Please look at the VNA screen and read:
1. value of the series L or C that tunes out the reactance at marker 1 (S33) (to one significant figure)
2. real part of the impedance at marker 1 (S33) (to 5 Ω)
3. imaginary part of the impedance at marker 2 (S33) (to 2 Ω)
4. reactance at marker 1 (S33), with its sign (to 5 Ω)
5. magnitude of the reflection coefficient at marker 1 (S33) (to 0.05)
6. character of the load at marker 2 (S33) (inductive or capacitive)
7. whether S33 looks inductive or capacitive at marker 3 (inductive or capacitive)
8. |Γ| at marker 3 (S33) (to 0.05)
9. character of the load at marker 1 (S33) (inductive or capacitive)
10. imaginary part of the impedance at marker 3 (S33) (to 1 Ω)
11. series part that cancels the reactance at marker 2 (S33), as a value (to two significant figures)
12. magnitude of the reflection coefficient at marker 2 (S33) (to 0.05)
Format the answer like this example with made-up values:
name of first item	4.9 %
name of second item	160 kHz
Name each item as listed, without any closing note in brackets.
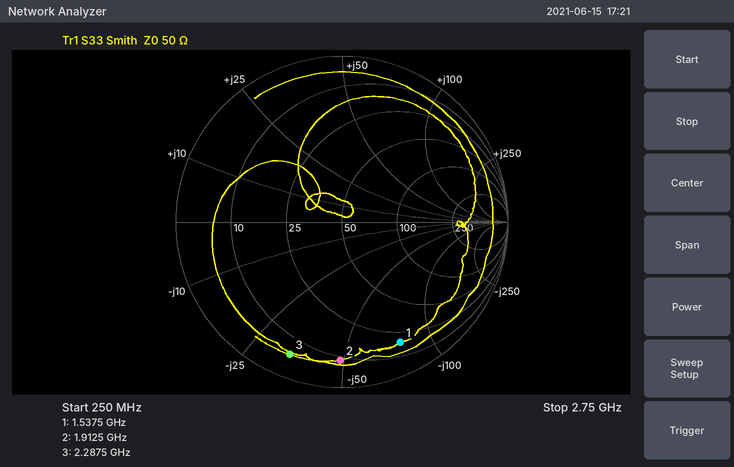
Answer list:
value of the series L or C that tunes out the reactance at marker 1 (S33)	8 nH
real part of the impedance at marker 1 (S33)	20 Ω
imaginary part of the impedance at marker 2 (S33)	-48 Ω
reactance at marker 1 (S33), with its sign	-75 Ω
magnitude of the reflection coefficient at marker 1 (S33)	0.80
character of the load at marker 2 (S33)	capacitive
whether S33 looks inductive or capacitive at marker 3	capacitive
|Γ| at marker 3 (S33)	0.85
character of the load at marker 1 (S33)	capacitive
imaginary part of the impedance at marker 3 (S33)	-34 Ω
series part that cancels the reactance at marker 2 (S33), as a value	4.0 nH
magnitude of the reflection coefficient at marker 2 (S33)	0.85
